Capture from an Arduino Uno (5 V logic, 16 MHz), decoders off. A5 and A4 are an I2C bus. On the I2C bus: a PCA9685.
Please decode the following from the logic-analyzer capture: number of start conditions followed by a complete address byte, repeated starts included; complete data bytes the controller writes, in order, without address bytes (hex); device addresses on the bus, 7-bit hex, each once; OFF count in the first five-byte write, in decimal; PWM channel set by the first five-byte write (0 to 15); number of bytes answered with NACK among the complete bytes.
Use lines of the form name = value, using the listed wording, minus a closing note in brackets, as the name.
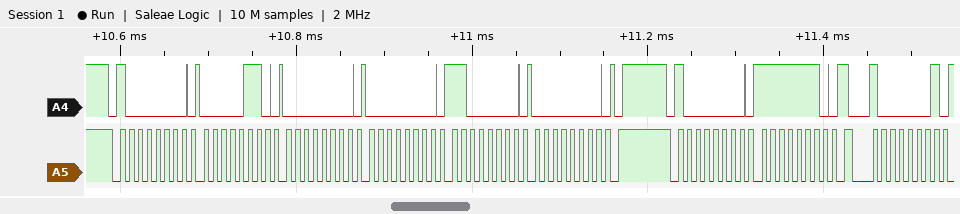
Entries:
number of start conditions followed by a complete address byte, repeated starts included = 3
complete data bytes the controller writes, in order, without address bytes = 06 00 00 C0 00 FE
device addresses on the bus, 7-bit hex, each once = 0x40
OFF count in the first five-byte write, in decimal = 192
PWM channel set by the first five-byte write = 0
number of bytes answered with NACK among the complete bytes = 0
